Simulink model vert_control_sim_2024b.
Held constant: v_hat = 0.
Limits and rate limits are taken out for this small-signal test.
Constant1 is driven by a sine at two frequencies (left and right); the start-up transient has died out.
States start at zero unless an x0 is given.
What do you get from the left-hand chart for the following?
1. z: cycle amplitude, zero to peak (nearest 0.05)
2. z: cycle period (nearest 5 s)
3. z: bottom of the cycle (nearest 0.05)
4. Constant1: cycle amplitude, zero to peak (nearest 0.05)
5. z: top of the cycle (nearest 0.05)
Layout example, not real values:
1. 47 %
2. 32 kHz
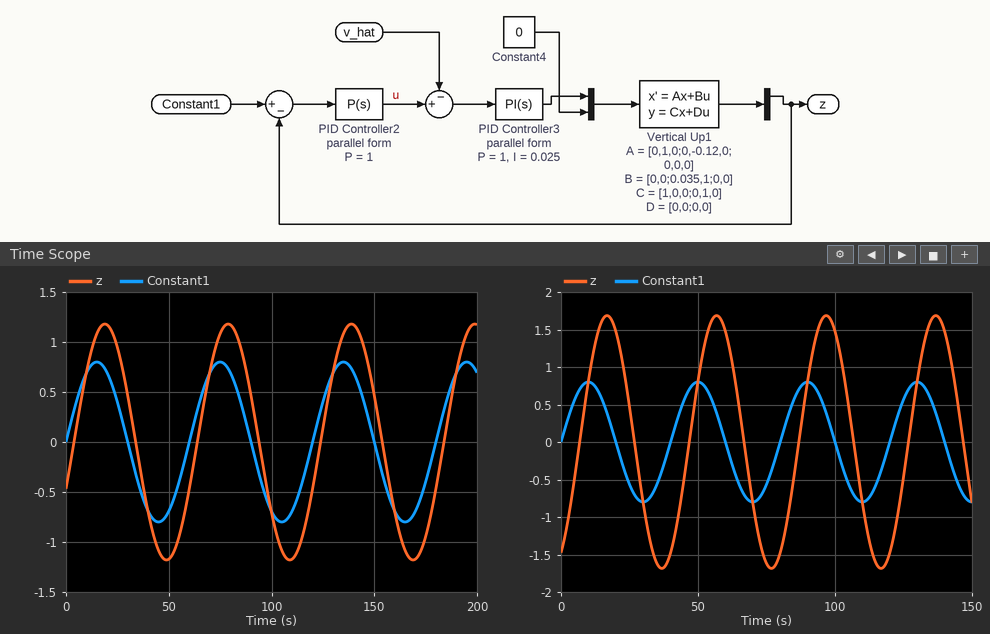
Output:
1. 1.20
2. 60 s
3. -1.20
4. 0.80
5. 1.20
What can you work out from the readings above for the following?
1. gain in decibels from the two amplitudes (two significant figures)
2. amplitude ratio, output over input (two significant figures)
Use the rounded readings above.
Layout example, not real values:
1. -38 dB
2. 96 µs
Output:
1. 3.5 dB
2. 1.5
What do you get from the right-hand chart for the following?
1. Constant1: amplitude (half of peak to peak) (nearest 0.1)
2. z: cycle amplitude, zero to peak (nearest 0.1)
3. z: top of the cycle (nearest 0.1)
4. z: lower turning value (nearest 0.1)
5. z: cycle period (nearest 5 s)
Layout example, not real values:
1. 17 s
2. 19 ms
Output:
1. 0.8
2. 1.7
3. 1.7
4. -1.7
5. 40 s
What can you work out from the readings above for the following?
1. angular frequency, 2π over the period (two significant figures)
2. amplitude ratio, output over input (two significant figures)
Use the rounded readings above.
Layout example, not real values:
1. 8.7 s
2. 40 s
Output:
1. 0.16 rad/s
2. 2.1
